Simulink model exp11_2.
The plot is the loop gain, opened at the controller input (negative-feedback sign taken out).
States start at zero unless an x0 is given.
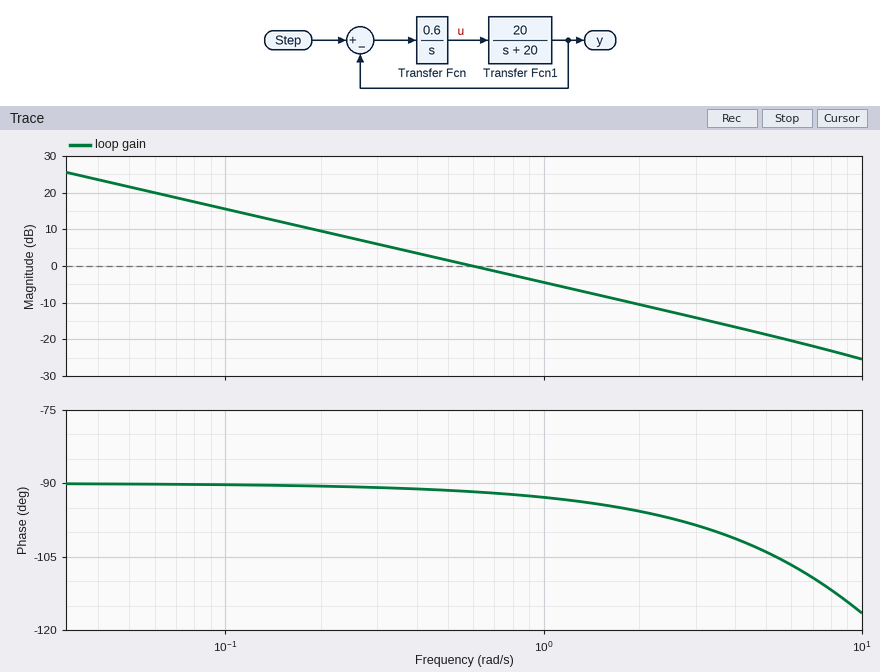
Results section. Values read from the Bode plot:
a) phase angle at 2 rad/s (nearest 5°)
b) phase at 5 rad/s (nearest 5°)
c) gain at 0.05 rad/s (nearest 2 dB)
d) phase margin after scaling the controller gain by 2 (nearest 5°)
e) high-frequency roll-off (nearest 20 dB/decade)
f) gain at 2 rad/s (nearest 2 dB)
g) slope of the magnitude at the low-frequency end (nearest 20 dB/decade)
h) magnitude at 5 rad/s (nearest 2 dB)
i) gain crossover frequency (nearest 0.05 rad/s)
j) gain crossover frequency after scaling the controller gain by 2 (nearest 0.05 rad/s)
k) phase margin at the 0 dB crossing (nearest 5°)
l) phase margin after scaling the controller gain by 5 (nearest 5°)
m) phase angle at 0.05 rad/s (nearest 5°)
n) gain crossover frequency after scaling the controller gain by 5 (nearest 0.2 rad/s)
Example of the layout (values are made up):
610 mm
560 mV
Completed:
-95°
-105°
22 dB
85°
-20 dB/decade
-10 dB
-20 dB/decade
-18 dB
0.60 rad/s
1.20 rad/s
90°
80°
-90°
3.0 rad/s
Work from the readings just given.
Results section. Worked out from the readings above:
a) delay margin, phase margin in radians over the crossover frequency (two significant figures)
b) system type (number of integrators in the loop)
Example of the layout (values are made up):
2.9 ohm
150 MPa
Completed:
2.6 s
1
